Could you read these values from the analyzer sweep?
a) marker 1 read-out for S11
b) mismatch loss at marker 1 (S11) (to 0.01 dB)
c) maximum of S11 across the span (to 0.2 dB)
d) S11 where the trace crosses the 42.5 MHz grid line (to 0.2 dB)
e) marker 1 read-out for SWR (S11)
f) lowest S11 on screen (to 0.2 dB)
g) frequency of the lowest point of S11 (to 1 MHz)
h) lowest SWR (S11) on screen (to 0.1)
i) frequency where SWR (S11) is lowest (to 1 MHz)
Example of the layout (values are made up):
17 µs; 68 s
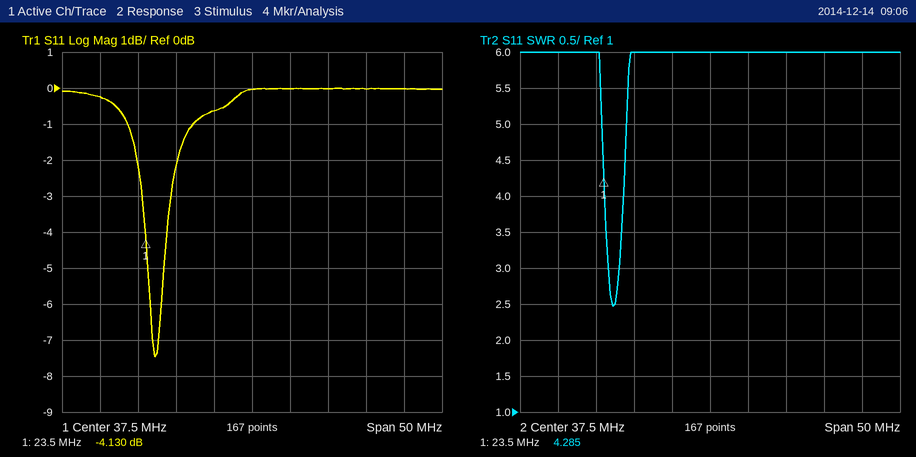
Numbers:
-4.130 dB; 2.12 dB; 0.0 dB; 0.0 dB; 4.285; -7.4 dB; 25 MHz; 2.5; 25 MHz
